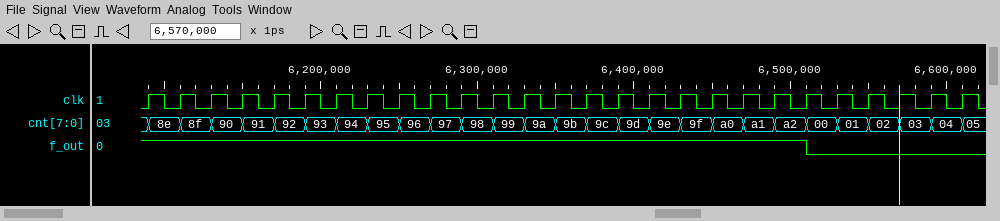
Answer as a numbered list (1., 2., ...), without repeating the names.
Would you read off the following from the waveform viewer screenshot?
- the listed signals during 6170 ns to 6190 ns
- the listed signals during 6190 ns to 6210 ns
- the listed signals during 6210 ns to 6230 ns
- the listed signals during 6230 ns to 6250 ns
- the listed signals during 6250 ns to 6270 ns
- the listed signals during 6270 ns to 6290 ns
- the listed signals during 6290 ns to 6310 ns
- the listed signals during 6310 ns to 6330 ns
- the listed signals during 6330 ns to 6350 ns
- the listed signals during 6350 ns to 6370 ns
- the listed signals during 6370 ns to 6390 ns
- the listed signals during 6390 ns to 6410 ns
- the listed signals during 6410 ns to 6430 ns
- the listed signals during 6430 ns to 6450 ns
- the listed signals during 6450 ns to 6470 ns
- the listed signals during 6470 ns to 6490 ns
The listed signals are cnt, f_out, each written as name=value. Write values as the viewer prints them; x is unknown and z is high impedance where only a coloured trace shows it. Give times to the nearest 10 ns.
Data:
1. cnt=92, f_out=1
2. cnt=93, f_out=1
3. cnt=94, f_out=1
4. cnt=95, f_out=1
5. cnt=96, f_out=1
6. cnt=97, f_out=1
7. cnt=98, f_out=1
8. cnt=99, f_out=1
9. cnt=9a, f_out=1
10. cnt=9b, f_out=1
11. cnt=9c, f_out=1
12. cnt=9d, f_out=1
13. cnt=9e, f_out=1
14. cnt=9f, f_out=1
15. cnt=a0, f_out=1
16. cnt=a1, f_out=1
